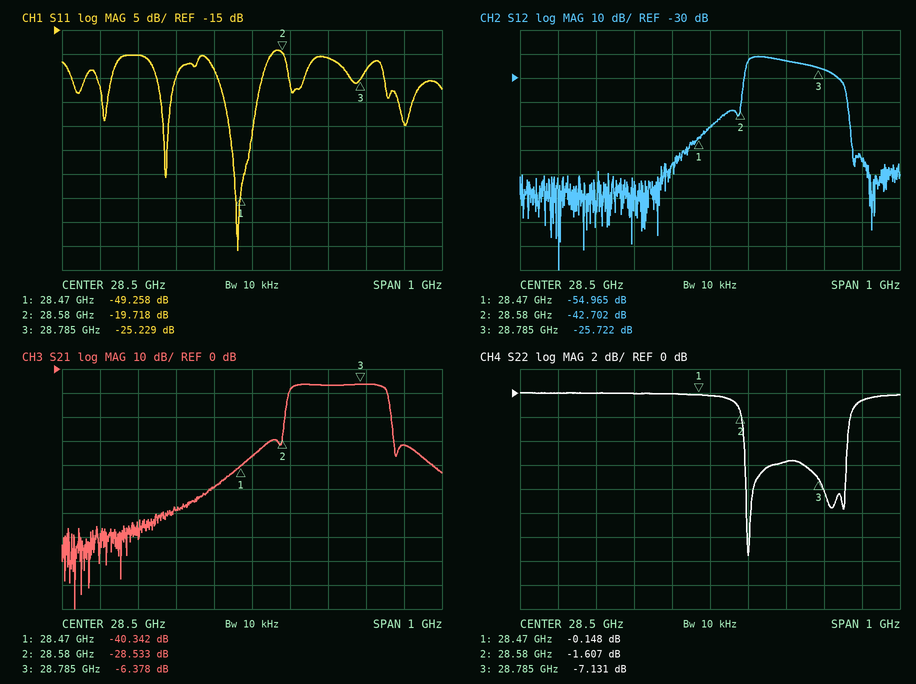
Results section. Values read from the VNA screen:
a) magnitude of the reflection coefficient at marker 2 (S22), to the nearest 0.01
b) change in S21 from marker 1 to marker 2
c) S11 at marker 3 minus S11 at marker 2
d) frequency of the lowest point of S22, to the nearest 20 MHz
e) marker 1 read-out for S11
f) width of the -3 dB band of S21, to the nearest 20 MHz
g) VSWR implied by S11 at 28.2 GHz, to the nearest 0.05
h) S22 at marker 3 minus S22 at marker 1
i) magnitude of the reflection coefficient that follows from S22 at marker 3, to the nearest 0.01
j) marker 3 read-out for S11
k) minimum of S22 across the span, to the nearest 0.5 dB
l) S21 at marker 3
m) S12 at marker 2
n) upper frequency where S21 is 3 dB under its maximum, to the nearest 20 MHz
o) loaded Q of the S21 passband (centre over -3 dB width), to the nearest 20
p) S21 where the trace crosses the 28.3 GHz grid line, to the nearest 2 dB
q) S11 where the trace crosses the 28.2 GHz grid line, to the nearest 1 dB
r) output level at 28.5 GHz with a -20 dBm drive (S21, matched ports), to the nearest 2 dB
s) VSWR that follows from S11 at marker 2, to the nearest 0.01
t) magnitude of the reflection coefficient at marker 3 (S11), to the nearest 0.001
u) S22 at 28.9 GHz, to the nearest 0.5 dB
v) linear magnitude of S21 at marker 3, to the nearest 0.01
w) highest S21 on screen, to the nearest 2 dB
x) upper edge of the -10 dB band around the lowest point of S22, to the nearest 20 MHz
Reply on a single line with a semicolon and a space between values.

0.83; 11.809 dB; -5.511 dB; 28.60 GHz; -49.258 dB; 260 MHz; 1.20; -6.983 dB; 0.44; -25.229 dB; -13.5 dB; -6.378 dB; -42.702 dB; 28.86 GHz; 120; -58 dB; -20 dB; -56 dBm; 1.23; 0.055; -0.5 dB; 0.48; -6 dB; 28.60 GHz
